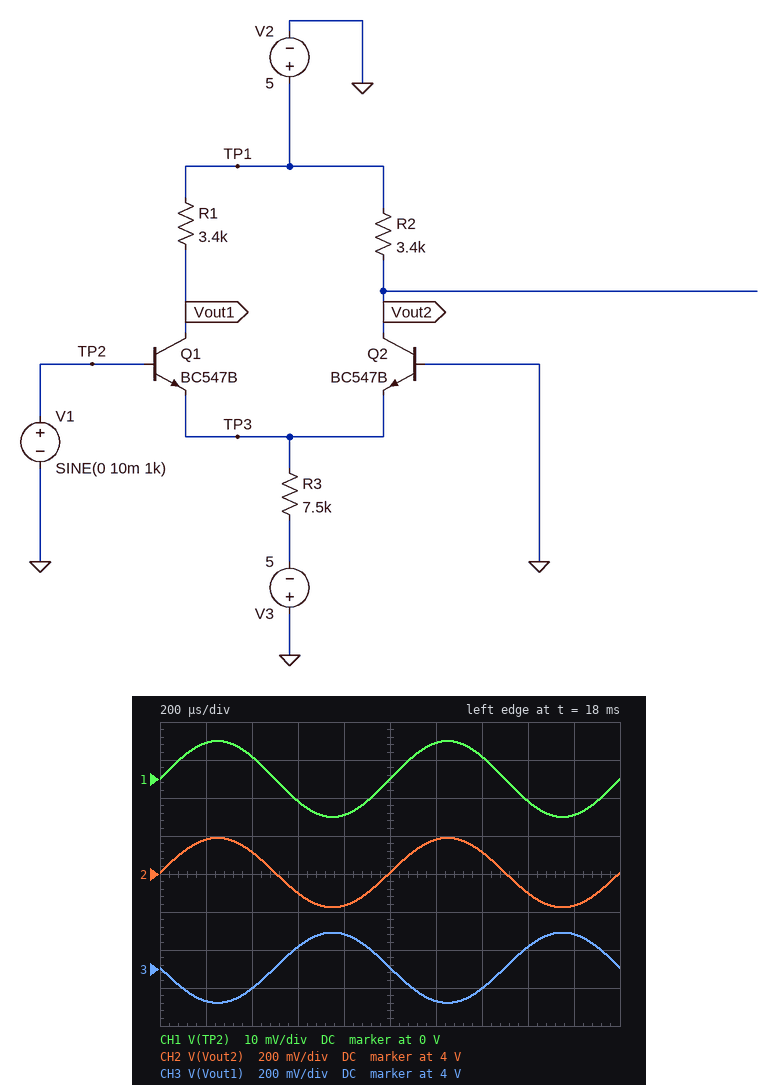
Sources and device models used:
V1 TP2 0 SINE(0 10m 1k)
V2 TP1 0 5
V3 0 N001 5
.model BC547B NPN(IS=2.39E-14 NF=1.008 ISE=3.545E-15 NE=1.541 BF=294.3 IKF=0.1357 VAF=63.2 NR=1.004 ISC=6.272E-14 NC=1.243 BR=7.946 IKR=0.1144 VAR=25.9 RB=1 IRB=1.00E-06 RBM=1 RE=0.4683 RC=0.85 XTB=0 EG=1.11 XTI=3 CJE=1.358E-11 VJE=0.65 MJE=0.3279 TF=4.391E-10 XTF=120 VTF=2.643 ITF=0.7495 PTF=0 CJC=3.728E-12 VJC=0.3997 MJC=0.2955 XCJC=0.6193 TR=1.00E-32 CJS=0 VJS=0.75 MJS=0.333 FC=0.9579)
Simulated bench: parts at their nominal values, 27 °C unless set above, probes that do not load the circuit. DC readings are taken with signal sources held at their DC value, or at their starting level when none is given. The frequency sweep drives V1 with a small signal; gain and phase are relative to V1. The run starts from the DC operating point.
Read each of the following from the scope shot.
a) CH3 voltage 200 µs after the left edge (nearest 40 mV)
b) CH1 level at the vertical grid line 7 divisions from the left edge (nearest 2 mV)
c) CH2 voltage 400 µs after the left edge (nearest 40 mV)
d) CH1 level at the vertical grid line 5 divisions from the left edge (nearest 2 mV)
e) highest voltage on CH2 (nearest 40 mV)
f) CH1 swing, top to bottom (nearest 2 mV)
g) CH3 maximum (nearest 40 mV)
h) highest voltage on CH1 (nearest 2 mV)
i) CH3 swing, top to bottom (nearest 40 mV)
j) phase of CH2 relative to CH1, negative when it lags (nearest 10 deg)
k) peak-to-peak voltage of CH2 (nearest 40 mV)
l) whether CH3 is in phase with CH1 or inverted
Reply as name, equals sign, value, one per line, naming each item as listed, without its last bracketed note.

CH3 voltage 200 µs after the left edge = 3.84 V
CH1 level at the vertical grid line 7 divisions from the left edge = 6 mV
CH2 voltage 400 µs after the left edge = 4.12 V
CH1 level at the vertical grid line 5 divisions from the left edge = 0 V
highest voltage on CH2 = 4.20 V
CH1 swing, top to bottom = 20 mV
CH3 maximum = 4.20 V
highest voltage on CH1 = 10 mV
CH3 swing, top to bottom = 360 mV
phase of CH2 relative to CH1, negative when it lags = 0 deg
peak-to-peak voltage of CH2 = 360 mV
whether CH3 is in phase with CH1 or inverted = inverted
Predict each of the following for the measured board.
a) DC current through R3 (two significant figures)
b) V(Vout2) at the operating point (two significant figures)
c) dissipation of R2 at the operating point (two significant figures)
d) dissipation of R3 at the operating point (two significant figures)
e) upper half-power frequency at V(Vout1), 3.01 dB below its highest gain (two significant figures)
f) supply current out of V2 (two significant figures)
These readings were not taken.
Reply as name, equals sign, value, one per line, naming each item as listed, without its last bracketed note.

DC current through R3 = 590 µA
V(Vout2) at the operating point = 4.0 V
dissipation of R2 at the operating point = 290 µW
dissipation of R3 at the operating point = 2.6 mW
upper half-power frequency at V(Vout1), 3.01 dB below its highest gain = 26 MHz
supply current out of V2 = 580 µA
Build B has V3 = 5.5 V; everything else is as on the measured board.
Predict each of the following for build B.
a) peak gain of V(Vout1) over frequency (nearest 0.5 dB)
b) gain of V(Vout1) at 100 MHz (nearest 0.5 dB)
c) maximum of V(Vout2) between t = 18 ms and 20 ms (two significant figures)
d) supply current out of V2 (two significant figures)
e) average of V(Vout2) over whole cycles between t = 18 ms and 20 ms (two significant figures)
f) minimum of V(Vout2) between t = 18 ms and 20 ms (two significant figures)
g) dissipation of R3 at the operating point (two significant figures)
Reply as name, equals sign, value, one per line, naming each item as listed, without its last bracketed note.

peak gain of V(Vout1) over frequency = 26.5 dB
gain of V(Vout1) at 100 MHz = 14.5 dB
maximum of V(Vout2) between t = 18 ms and 20 ms = 4.1 V
supply current out of V2 = 650 µA
average of V(Vout2) over whole cycles between t = 18 ms and 20 ms = 3.9 V
minimum of V(Vout2) between t = 18 ms and 20 ms = 3.7 V
dissipation of R3 at the operating point = 3.2 mW
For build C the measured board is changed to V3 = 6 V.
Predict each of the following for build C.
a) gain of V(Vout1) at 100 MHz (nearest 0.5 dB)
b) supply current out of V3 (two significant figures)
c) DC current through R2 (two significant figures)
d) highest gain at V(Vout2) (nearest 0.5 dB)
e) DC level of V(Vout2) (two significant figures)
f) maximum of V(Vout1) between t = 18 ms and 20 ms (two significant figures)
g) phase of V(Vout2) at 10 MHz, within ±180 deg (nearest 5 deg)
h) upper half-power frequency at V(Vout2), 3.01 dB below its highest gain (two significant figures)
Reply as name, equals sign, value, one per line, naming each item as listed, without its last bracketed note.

gain of V(Vout1) at 100 MHz = 15.0 dB
supply current out of V3 = 720 µA
DC current through R2 = 360 µA
highest gain at V(Vout2) = 27.0 dB
DC level of V(Vout2) = 3.8 V
maximum of V(Vout1) between t = 18 ms and 20 ms = 4.0 V
phase of V(Vout2) at 10 MHz, within ±180 deg = -20 deg
upper half-power frequency at V(Vout2), 3.01 dB below its highest gain = 25 MHz
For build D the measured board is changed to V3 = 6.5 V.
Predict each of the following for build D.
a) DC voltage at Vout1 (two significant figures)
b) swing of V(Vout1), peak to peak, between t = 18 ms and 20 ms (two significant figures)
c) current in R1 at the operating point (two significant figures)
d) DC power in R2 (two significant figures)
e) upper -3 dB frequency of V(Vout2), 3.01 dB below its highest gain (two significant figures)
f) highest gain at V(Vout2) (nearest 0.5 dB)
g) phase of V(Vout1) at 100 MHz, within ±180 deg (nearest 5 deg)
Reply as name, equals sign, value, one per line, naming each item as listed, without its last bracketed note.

DC voltage at Vout1 = 3.7 V
swing of V(Vout1), peak to peak, between t = 18 ms and 20 ms = 490 mV
current in R1 at the operating point = 390 µA
DC power in R2 = 520 µW
upper -3 dB frequency of V(Vout2), 3.01 dB below its highest gain = 25 MHz
highest gain at V(Vout2) = 28.0 dB
phase of V(Vout1) at 100 MHz, within ±180 deg = 95 deg
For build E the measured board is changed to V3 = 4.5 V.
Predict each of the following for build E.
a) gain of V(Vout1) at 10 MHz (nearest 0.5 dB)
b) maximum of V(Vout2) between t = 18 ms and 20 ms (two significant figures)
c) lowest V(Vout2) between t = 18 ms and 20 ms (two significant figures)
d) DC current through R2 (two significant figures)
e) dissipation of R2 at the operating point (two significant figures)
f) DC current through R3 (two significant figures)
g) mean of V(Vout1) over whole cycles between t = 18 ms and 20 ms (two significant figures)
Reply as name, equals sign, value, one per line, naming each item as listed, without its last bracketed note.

gain of V(Vout1) at 10 MHz = 24.0 dB
maximum of V(Vout2) between t = 18 ms and 20 ms = 4.3 V
lowest V(Vout2) between t = 18 ms and 20 ms = 4.0 V
DC current through R2 = 260 µA
dissipation of R2 at the operating point = 230 µW
DC current through R3 = 520 µA
mean of V(Vout1) over whole cycles between t = 18 ms and 20 ms = 4.1 V
